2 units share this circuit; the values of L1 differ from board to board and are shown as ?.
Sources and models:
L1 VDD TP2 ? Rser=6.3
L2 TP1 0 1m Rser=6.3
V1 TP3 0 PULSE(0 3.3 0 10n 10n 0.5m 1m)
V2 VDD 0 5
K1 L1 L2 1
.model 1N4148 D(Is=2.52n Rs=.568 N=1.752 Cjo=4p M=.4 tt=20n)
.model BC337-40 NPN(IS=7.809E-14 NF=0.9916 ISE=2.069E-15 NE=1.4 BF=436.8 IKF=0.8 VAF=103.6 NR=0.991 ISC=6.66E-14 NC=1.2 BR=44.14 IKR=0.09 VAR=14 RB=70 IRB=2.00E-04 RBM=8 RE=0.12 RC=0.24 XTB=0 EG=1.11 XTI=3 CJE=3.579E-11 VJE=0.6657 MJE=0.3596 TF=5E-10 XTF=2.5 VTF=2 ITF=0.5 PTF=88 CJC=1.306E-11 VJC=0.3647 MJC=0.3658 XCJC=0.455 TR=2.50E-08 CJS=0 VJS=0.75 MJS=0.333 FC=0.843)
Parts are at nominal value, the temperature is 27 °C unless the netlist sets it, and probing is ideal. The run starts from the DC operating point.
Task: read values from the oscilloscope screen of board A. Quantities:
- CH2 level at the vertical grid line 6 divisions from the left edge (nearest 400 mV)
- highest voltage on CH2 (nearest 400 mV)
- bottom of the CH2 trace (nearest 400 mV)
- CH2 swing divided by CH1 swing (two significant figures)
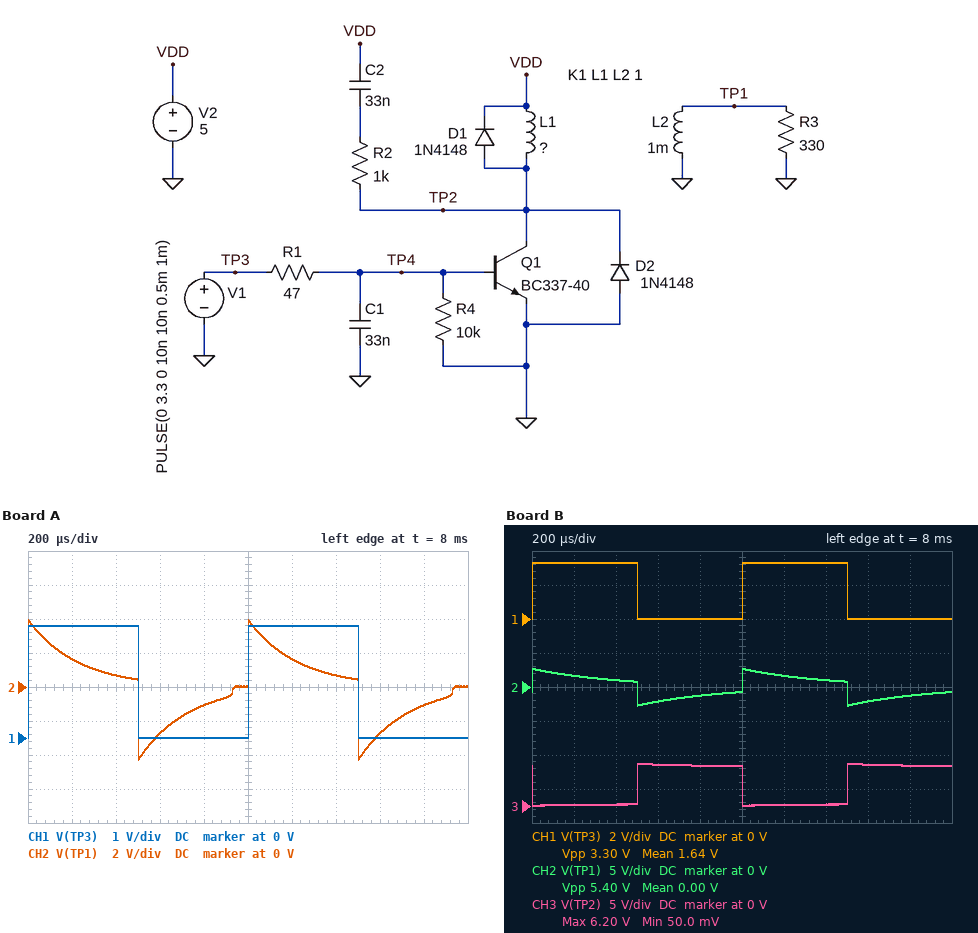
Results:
1.6 V
4.0 V
-4.4 V
2.5
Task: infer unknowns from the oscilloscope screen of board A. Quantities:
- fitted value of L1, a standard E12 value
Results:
1.5 mH
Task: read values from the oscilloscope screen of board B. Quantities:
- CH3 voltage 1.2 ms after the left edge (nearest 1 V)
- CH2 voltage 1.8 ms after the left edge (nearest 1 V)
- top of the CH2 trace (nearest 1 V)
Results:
0 V
-1 V
3 V
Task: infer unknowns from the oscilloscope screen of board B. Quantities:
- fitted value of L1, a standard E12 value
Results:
2.7 mH
